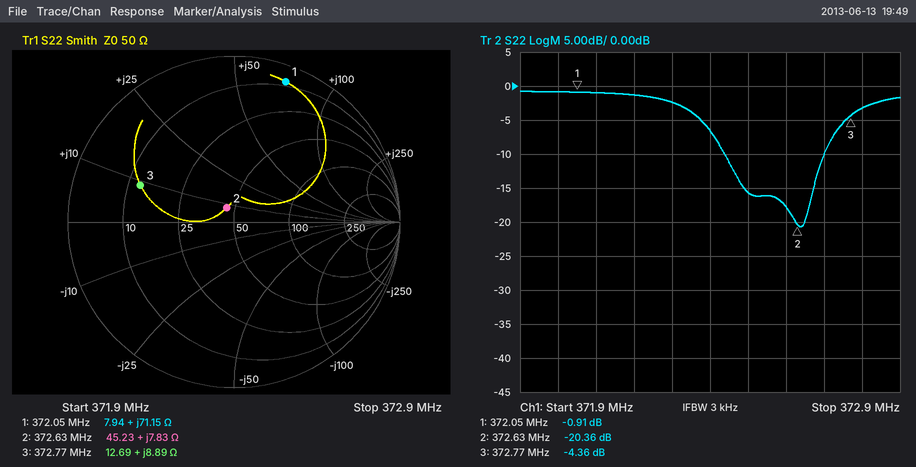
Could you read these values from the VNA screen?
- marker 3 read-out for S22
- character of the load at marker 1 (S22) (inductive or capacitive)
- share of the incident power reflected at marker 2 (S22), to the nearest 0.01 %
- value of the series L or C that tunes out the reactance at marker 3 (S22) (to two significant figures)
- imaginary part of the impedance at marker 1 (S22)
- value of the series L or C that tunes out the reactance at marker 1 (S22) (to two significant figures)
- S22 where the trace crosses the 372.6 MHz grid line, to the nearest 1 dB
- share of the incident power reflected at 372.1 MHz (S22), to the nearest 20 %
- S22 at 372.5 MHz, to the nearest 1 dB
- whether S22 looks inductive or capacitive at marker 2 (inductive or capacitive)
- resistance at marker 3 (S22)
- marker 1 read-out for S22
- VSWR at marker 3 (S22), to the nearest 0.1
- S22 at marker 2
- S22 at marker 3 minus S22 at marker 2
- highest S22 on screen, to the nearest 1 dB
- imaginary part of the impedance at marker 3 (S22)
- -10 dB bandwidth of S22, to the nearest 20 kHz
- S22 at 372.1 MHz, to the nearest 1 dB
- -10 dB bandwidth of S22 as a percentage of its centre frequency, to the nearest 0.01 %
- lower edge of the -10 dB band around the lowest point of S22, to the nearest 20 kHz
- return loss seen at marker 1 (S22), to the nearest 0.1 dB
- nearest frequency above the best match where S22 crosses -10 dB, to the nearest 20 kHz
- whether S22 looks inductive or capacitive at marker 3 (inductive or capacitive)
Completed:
-4.36 dB
inductive
0.92 %
48 pF
+71.15 Ω
6.0 pF
-18 dB
80 %
-16 dB
inductive
12.69 Ω
-0.91 dB
4.1
-20.36 dB
16.00 dB
-1 dB
+8.89 Ω
260 kHz
-1 dB
0.07 %
372.44 MHz
0.9 dB
372.70 MHz
inductive
